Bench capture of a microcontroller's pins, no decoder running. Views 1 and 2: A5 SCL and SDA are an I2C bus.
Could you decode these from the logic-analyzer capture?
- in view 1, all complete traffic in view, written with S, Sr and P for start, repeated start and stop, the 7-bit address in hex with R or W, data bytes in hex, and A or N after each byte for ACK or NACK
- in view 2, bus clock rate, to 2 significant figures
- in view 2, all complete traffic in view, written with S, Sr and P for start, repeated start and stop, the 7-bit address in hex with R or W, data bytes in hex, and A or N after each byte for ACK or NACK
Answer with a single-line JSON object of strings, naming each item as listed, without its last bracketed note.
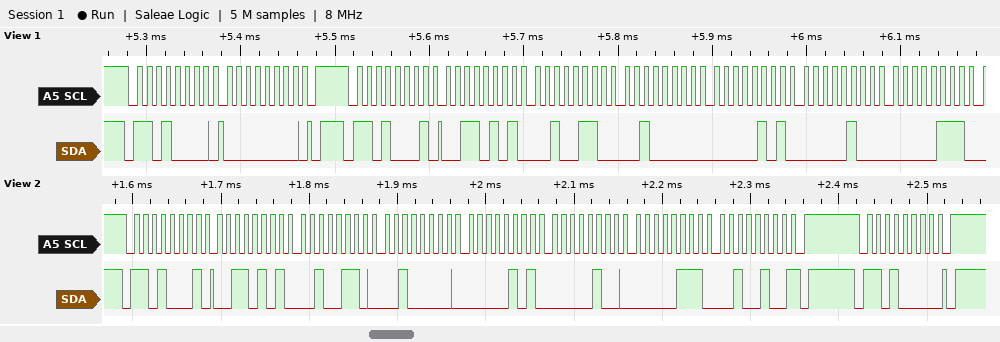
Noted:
{"in view 1, all complete traffic in view, written with S, Sr and P for start, repeated start and stop, the 7-bit address in hex with R or W, data bytes in hex, and A or N after each byte for ACK or NACK": "S 68W A 00 A P S 68R A 35 A 26 A 20 A 05 A 04 A 07 A", "in view 2, bus clock rate, to 2 significant figures": "100 kHz", "in view 2, all complete traffic in view, written with S, Sr and P for start, repeated start and stop, the 7-bit address in hex with R or W, data bytes in hex, and A or N after each byte for ACK or NACK": "S 68R A 35 A 26 A 20 A 05 A 04 A 07 A 24 N P S 68W A P"}
